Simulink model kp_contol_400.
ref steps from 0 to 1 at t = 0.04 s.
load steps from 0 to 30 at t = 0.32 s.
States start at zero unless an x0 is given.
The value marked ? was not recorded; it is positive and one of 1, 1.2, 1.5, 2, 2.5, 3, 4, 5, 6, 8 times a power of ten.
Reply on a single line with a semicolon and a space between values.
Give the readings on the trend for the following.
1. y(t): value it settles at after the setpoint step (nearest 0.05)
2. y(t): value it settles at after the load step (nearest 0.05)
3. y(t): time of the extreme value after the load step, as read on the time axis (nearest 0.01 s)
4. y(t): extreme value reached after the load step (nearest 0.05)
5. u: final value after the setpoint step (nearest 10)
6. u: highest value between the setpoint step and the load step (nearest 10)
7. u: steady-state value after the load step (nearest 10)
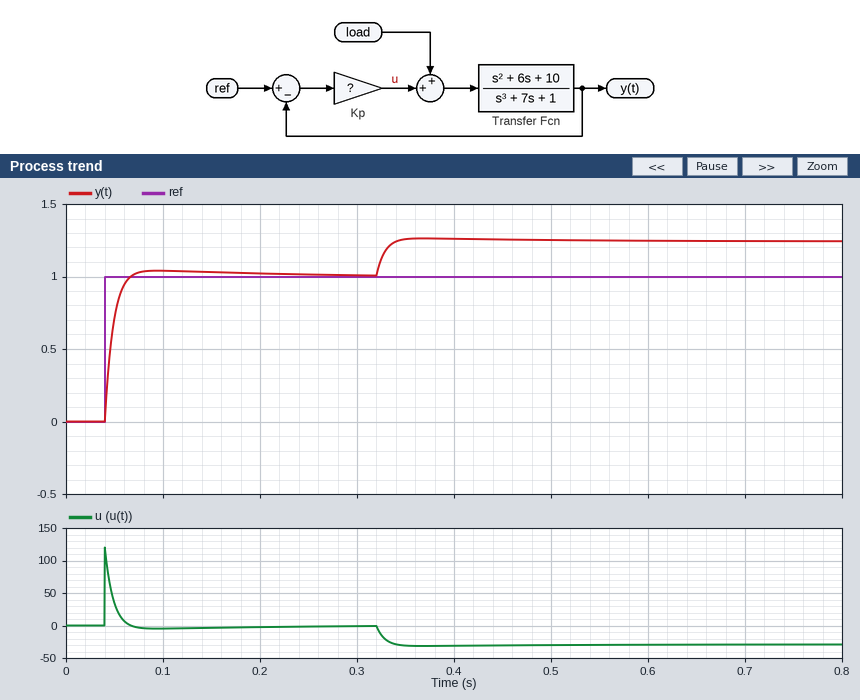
1.00; 1.25; 0.37 s; 1.25; 0; 120; -30
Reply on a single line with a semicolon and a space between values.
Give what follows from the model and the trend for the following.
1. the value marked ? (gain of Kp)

120
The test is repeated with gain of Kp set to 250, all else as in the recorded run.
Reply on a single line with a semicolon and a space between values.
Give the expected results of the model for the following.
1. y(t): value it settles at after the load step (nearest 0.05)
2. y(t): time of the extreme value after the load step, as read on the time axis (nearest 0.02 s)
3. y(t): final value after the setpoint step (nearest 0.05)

1.10; 0.34 s; 1.00
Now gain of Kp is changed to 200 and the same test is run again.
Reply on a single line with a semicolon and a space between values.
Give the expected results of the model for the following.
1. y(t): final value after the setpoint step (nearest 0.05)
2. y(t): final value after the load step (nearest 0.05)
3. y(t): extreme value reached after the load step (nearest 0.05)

1.00; 1.15; 1.15
